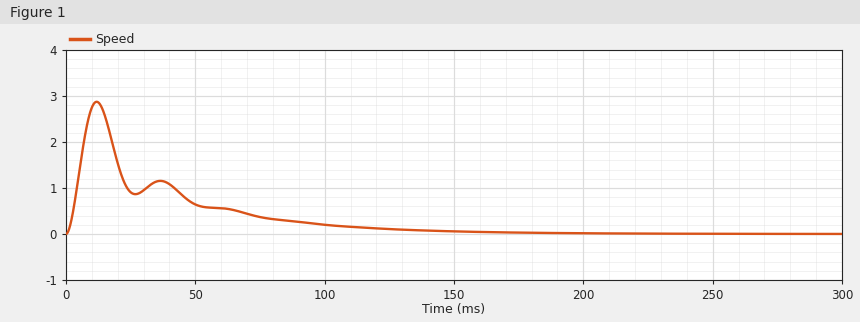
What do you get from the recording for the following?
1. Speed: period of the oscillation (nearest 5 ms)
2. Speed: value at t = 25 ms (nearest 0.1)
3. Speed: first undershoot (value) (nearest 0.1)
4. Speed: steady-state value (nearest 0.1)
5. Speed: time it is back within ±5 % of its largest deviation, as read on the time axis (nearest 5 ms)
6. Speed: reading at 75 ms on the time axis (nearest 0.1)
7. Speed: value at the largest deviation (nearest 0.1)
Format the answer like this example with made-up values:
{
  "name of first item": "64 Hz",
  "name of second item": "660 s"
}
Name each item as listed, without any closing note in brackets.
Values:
{
  "Speed: period of the oscillation": "25 ms",
  "Speed: value at t = 25 ms": "0.9",
  "Speed: first undershoot (value)": "0.9",
  "Speed: steady-state value": "0.0",
  "Speed: time it is back within ±5 % of its largest deviation, as read on the time axis": "115 ms",
  "Speed: reading at 75 ms on the time axis": "0.4",
  "Speed: value at the largest deviation": "2.9"
}
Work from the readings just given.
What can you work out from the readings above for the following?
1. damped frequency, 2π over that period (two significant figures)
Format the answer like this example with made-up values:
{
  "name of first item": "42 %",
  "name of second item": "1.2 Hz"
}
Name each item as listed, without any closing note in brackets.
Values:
{
  "damped frequency, 2π over that period": "0.25 rad/ms"
}
